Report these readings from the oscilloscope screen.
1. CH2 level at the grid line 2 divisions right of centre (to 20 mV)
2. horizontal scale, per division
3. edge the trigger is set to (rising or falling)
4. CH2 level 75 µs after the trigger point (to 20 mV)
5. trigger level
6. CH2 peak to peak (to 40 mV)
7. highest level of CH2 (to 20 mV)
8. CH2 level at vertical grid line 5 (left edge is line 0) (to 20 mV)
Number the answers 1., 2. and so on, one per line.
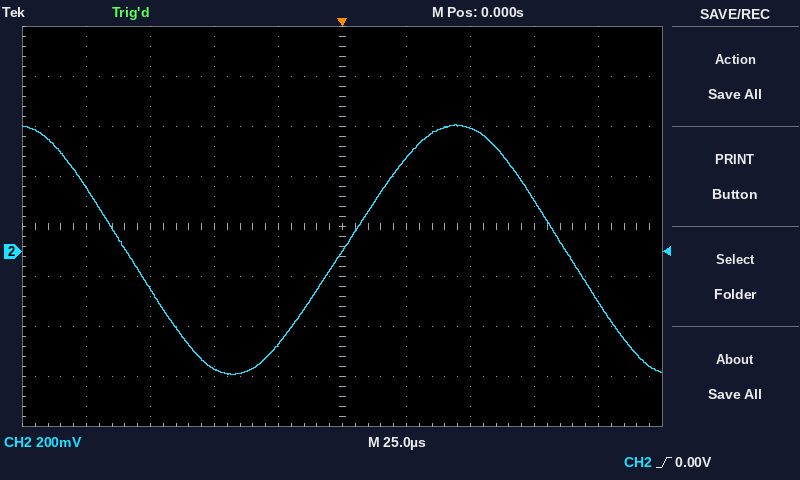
1. 500 mV
2. 25 µs
3. rising
4. 200 mV
5. 0.00 V
6. 1.00 V
7. 500 mV
8. 0 mV
